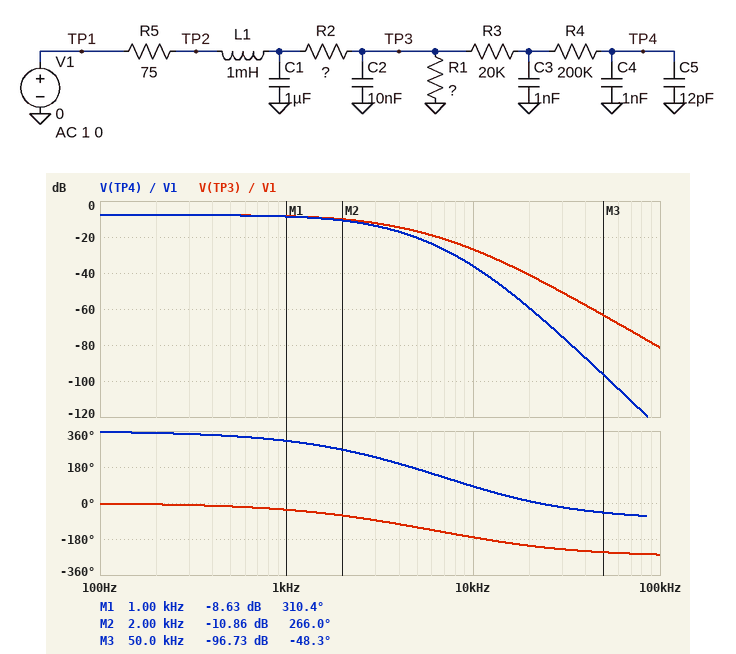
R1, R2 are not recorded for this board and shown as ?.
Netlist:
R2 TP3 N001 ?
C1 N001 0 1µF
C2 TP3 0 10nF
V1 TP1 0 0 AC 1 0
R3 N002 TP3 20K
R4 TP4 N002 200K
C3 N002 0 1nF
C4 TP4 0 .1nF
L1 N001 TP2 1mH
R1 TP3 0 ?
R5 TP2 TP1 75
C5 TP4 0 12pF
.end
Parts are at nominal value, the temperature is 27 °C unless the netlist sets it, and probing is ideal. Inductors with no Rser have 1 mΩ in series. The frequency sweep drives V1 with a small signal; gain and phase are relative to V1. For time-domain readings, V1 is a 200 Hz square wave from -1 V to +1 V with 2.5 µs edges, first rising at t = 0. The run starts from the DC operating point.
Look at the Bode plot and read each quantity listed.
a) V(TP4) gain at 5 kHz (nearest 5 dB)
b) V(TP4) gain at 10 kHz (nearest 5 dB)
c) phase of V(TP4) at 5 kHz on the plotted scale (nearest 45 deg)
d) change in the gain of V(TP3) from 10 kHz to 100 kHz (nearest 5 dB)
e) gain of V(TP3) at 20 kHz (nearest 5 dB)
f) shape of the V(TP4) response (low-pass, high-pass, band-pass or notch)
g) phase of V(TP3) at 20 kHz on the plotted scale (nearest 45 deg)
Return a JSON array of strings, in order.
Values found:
["-20 dB", "-35 dB", "180 deg", "-55 dB", "-40 dB", "low-pass", "-225 deg"]
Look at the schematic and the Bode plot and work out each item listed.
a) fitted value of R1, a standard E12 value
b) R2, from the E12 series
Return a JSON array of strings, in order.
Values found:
["3.3 kΩ", "4.7 kΩ"]
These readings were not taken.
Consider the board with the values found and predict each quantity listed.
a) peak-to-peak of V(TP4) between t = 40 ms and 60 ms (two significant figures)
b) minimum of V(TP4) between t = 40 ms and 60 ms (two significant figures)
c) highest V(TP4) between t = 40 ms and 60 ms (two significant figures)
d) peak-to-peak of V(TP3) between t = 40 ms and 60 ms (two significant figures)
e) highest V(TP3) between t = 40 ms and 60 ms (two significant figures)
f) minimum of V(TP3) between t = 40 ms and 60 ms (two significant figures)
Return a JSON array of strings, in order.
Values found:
["820 mV", "-410 mV", "410 mV", "820 mV", "410 mV", "-410 mV"]
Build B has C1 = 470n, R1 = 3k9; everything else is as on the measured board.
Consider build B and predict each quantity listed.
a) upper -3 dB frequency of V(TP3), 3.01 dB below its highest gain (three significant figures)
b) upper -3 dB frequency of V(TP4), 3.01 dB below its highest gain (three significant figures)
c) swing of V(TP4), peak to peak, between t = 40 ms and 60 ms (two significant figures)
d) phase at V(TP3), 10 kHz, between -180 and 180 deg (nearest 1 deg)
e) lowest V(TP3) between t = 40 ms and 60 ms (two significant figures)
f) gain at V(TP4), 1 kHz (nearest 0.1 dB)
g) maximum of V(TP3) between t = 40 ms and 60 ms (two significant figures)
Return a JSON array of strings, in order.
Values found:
["4.41 kHz", "3.03 kHz", "900 mV", "-163 deg", "-450 mV", "-7.3 dB", "450 mV"]
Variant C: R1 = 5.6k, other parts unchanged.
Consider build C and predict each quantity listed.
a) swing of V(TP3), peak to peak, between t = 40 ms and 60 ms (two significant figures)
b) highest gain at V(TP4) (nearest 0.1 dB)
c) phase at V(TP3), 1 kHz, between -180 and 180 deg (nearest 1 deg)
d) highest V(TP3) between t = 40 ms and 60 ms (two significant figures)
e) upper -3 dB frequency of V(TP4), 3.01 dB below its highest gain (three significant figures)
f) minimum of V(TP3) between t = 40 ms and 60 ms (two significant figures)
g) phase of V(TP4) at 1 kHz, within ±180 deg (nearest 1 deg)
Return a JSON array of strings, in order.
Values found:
["1.1 V", "-5.4 dB", "-36 deg", "540 mV", "1.89 kHz", "-540 mV", "-52 deg"]
